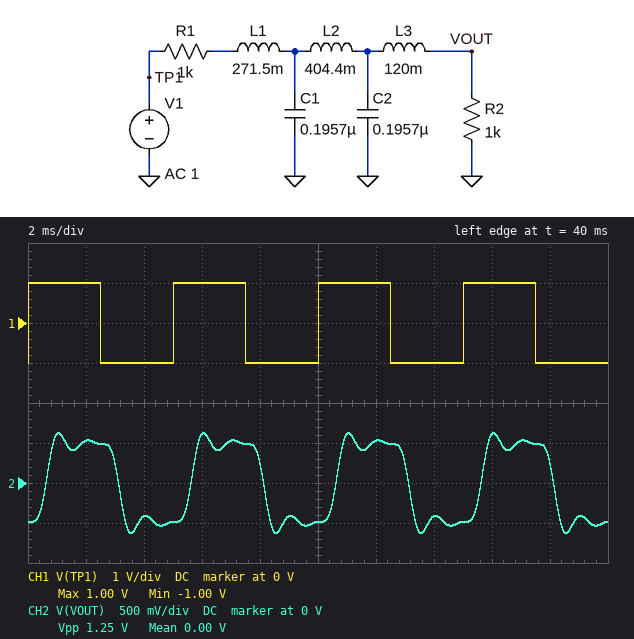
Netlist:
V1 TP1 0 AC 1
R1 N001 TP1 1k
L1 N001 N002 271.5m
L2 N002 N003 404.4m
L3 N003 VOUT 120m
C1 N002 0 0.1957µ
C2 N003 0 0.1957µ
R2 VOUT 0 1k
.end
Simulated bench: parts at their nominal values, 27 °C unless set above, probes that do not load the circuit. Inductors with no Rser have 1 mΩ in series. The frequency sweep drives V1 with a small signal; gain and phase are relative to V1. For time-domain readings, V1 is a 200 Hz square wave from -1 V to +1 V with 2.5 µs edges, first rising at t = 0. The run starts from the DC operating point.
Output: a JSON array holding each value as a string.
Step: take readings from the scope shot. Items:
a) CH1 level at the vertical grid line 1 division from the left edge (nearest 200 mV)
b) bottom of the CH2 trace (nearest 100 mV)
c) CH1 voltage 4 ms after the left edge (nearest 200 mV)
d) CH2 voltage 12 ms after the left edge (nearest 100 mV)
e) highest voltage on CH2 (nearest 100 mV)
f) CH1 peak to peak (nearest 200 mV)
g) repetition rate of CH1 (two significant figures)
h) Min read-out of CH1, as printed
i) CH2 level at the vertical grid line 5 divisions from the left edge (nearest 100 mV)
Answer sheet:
["1.0 V", "-600 mV", "-1.0 V", "500 mV", "600 mV", "2.0 V", "200 Hz", "-1.00 V", "-500 mV"]
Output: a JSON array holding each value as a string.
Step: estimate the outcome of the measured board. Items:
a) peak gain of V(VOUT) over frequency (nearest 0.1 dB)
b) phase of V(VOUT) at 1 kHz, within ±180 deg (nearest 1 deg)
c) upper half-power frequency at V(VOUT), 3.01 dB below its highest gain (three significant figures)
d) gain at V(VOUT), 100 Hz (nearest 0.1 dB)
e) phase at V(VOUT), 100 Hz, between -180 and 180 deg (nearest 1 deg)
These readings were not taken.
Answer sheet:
["-6.0 dB", "110 deg", "1.05 kHz", "-6.1 dB", "-21 deg"]
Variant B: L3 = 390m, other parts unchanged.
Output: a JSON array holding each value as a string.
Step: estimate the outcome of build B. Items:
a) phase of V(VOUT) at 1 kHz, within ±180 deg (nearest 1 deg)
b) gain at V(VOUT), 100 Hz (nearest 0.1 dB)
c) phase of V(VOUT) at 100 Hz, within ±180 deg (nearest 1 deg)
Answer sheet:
["52 deg", "-6.2 dB", "-26 deg"]
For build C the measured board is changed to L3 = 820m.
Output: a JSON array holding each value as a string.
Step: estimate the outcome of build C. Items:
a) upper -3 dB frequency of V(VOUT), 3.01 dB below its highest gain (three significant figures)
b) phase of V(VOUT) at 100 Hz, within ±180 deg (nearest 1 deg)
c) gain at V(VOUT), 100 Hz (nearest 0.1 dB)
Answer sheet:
["585 Hz", "-33 deg", "-6.5 dB"]
